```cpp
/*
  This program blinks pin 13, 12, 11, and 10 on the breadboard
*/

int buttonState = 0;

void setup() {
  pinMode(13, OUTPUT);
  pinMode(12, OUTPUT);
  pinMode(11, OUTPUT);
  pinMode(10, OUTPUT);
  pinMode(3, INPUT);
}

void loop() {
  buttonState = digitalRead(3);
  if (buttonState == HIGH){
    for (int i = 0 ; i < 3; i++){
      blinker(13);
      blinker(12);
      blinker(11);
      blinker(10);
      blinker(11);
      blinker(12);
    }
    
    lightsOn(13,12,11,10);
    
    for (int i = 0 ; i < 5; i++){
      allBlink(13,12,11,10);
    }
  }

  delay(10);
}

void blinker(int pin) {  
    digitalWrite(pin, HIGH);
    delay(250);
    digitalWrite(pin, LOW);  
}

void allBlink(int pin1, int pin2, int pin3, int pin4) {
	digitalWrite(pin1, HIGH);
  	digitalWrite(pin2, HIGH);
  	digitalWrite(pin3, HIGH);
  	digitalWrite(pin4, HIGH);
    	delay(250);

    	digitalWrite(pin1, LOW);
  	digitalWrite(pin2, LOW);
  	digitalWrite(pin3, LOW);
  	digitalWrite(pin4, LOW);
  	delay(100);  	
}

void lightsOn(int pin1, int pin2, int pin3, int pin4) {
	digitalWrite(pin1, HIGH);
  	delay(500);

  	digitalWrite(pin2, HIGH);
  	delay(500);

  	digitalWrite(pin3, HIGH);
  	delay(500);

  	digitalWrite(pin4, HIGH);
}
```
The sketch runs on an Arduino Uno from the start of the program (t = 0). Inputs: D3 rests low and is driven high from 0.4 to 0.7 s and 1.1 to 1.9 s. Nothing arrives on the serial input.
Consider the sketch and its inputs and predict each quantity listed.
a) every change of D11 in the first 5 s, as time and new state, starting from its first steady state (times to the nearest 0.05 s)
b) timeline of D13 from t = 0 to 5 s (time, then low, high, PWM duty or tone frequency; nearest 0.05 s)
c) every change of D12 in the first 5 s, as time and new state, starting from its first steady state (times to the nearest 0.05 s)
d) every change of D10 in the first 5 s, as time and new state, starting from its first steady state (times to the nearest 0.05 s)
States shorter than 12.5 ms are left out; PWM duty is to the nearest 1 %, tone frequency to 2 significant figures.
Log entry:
0 s low; 0.9 s high; 1.15 s low; 1.4 s high; 1.65 s low; 2.4 s high; 2.65 s low; 2.9 s high; 3.15 s low; 3.9 s high; 4.15 s low; 4.4 s high; 4.65 s low
0 s low; 0.4 s high; 0.65 s low; 1.9 s high; 2.15 s low; 3.4 s high; 3.65 s low; 4.9 s high
0 s low; 0.65 s high; 0.9 s low; 1.65 s high; 1.9 s low; 2.15 s high; 2.4 s low; 3.15 s high; 3.4 s low; 3.65 s high; 3.9 s low; 4.65 s high; 4.9 s low
0 s low; 1.15 s high; 1.4 s low; 2.65 s high; 2.9 s low; 4.15 s high; 4.4 s low
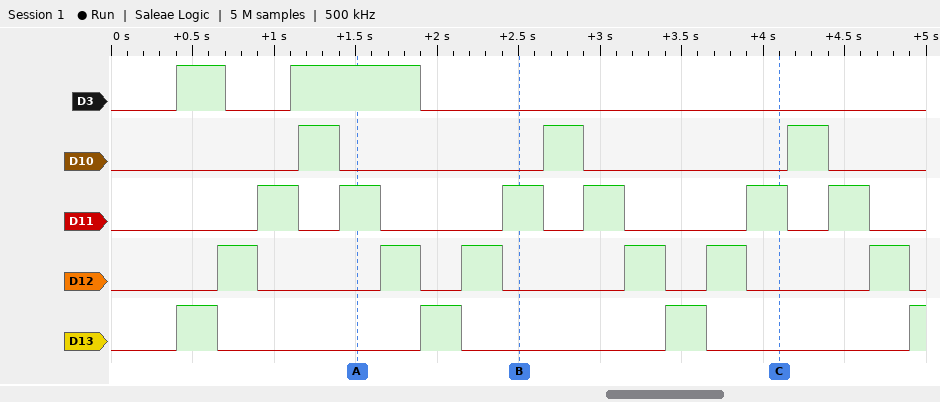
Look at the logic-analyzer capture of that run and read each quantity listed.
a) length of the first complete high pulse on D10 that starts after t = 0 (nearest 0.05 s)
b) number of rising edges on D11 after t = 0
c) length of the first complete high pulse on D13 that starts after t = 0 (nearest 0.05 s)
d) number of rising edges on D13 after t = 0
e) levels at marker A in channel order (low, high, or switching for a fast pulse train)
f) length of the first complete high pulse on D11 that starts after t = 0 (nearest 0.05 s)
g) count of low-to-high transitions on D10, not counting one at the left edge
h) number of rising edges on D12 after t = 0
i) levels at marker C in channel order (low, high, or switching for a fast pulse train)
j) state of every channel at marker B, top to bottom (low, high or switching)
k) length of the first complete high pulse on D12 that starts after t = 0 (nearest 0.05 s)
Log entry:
0.25 s
6
0.25 s
4
D3 high, D10 low, D11 high, D12 low, D13 low
0.25 s
3
6
D3 low, D10 low, D11 high, D12 low, D13 low
D3 low, D10 low, D11 high, D12 low, D13 low
0.25 s
